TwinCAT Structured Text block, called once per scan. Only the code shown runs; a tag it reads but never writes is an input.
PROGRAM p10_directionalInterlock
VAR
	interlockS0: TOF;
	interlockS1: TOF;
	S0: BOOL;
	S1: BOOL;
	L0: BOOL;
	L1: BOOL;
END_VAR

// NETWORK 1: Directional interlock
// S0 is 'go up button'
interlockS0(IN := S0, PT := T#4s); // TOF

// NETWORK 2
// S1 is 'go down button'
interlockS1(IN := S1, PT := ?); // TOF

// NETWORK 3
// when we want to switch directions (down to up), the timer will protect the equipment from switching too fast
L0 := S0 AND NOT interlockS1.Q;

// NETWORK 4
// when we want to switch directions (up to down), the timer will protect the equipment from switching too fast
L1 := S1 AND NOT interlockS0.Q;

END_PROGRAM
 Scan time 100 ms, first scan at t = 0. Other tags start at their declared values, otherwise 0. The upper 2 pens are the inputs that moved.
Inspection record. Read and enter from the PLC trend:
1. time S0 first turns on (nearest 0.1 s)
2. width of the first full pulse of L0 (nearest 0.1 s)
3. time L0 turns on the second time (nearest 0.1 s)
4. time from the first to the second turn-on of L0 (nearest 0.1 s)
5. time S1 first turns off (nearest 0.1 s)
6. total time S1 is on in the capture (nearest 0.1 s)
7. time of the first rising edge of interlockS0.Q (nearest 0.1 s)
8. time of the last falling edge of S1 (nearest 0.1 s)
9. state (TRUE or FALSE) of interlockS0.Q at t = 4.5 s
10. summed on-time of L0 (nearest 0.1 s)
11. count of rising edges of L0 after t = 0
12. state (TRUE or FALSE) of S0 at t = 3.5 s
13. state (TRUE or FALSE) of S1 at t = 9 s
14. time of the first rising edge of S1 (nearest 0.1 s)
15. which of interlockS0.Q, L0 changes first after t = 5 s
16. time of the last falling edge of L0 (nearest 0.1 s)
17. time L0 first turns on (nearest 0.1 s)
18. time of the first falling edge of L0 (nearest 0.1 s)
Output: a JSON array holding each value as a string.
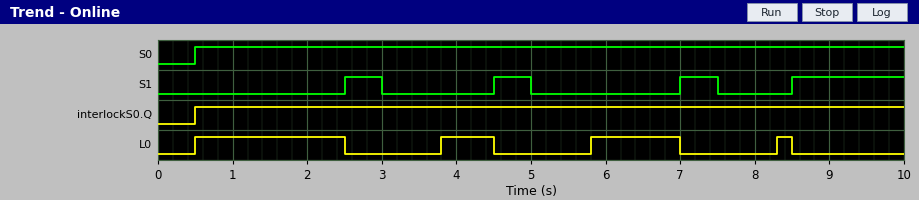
["0.5 s", "2.0 s", "3.8 s", "3.3 s", "3.0 s", "3.0 s", "0.5 s", "7.5 s", "TRUE", "4.1 s", "4", "TRUE", "TRUE", "2.5 s", "L0", "8.5 s", "0.5 s", "2.5 s"]
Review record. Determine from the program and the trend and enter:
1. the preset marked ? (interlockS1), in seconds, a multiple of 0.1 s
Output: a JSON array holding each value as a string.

["0.8 s"]
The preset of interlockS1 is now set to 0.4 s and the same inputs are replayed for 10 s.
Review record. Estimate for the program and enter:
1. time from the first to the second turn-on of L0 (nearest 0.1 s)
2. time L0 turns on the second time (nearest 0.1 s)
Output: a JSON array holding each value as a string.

["2.9 s", "3.4 s"]
